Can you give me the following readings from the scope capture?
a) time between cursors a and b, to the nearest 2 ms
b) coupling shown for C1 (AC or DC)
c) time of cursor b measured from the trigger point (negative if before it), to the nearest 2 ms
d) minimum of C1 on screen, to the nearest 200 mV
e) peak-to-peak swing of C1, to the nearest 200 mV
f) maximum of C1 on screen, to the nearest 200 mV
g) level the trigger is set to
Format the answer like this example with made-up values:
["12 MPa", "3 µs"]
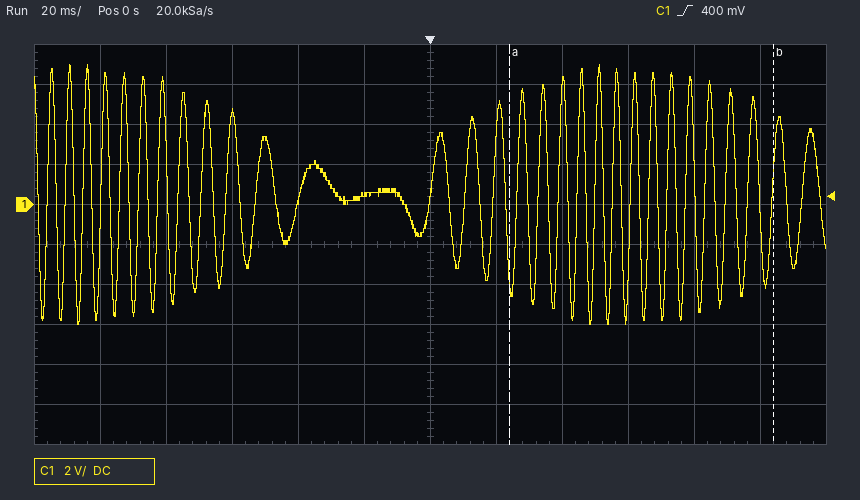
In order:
["80 ms", "DC", "+104 ms", "-6.0 V", "13.0 V", "7.0 V", "400 mV"]
